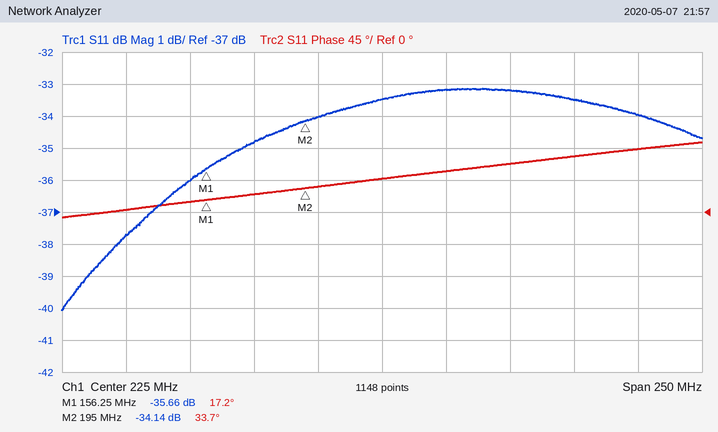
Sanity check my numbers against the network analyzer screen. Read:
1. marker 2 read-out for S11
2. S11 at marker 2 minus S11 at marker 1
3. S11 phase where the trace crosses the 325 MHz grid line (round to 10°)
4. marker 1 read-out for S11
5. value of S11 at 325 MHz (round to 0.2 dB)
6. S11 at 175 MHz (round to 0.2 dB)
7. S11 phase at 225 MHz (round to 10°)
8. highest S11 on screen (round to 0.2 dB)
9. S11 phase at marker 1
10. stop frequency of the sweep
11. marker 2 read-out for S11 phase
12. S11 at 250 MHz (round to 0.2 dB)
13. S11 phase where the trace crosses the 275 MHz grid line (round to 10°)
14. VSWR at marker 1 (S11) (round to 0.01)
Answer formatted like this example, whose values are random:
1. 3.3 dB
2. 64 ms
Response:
1. -34.14 dB
2. 1.52 dB
3. 90°
4. -35.66 dB
5. -34.0 dB
6. -34.8 dB
7. 50°
8. -33.2 dB
9. 17.2°
10. 350 MHz
11. 33.7°
12. -33.2 dB
13. 70°
14. 1.03
